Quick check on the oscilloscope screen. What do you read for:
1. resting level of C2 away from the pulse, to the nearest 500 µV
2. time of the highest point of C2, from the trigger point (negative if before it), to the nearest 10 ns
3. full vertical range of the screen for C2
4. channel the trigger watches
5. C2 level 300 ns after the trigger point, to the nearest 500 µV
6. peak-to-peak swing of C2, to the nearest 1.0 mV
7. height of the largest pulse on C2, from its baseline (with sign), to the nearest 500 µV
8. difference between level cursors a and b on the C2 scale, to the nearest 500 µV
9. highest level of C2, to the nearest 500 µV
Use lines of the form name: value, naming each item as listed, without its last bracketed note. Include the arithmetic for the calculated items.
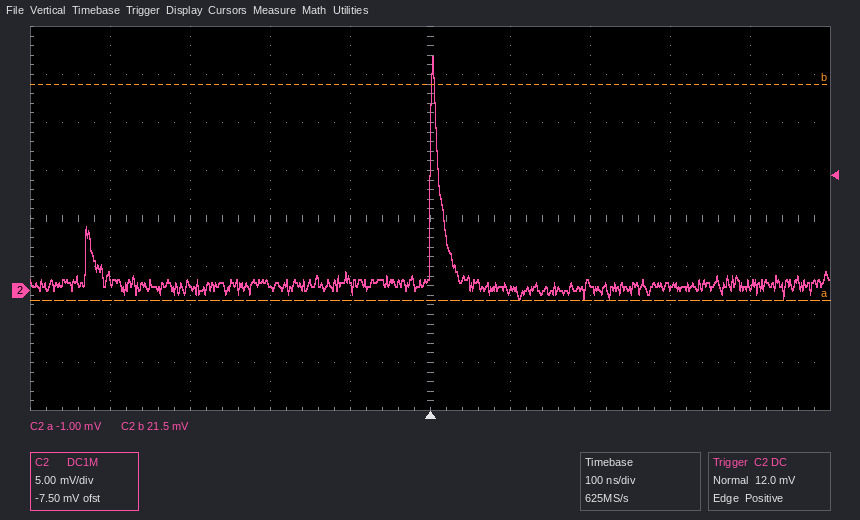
resting level of C2 away from the pulse, to the nearest 500 µV: 500 µV
time of the highest point of C2, from the trigger point (negative if before it), to the nearest 10 ns: 0 ns
full vertical range of the screen for C2: 40 mV
channel the trigger watches: C2
C2 level 300 ns after the trigger point, to the nearest 500 µV: 500 µV
peak-to-peak swing of C2, to the nearest 1.0 mV: 25.0 mV
height of the largest pulse on C2, from its baseline (with sign), to the nearest 500 µV: 24.5 mV − (500 µV) = +24.0 mV
difference between level cursors a and b on the C2 scale, to the nearest 500 µV: 22.5 mV
highest level of C2, to the nearest 500 µV: 24.5 mV
